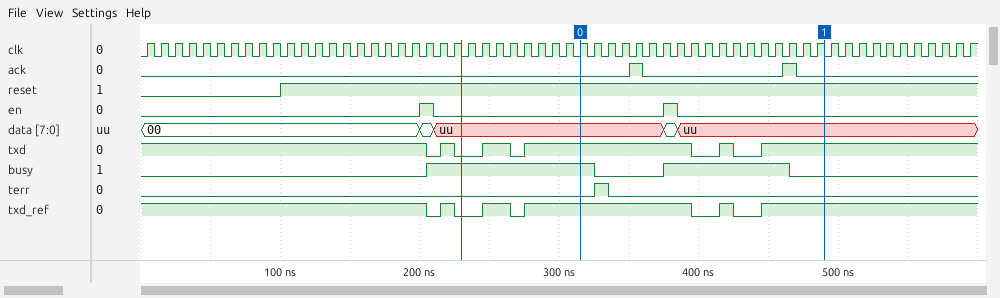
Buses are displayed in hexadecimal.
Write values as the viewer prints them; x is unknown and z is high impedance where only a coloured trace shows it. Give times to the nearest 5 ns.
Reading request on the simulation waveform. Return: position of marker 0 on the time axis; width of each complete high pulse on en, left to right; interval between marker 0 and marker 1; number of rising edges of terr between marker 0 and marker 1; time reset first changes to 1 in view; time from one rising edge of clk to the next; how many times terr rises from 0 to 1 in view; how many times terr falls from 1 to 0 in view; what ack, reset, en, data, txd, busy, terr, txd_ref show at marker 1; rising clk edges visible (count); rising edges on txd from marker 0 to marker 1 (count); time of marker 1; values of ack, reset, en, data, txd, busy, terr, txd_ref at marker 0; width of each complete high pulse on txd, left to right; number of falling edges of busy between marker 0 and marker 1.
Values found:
315 ns
10 ns, 10 ns
175 ns
1
100 ns
10 ns
1
1
ack=0, reset=1, en=0, data=uu, txd=1, busy=0, terr=0, txd_ref=1
60
2
490 ns
ack=0, reset=1, en=0, data=uu, txd=1, busy=1, terr=0, txd_ref=1
10 ns, 20 ns, 120 ns, 10 ns
2
